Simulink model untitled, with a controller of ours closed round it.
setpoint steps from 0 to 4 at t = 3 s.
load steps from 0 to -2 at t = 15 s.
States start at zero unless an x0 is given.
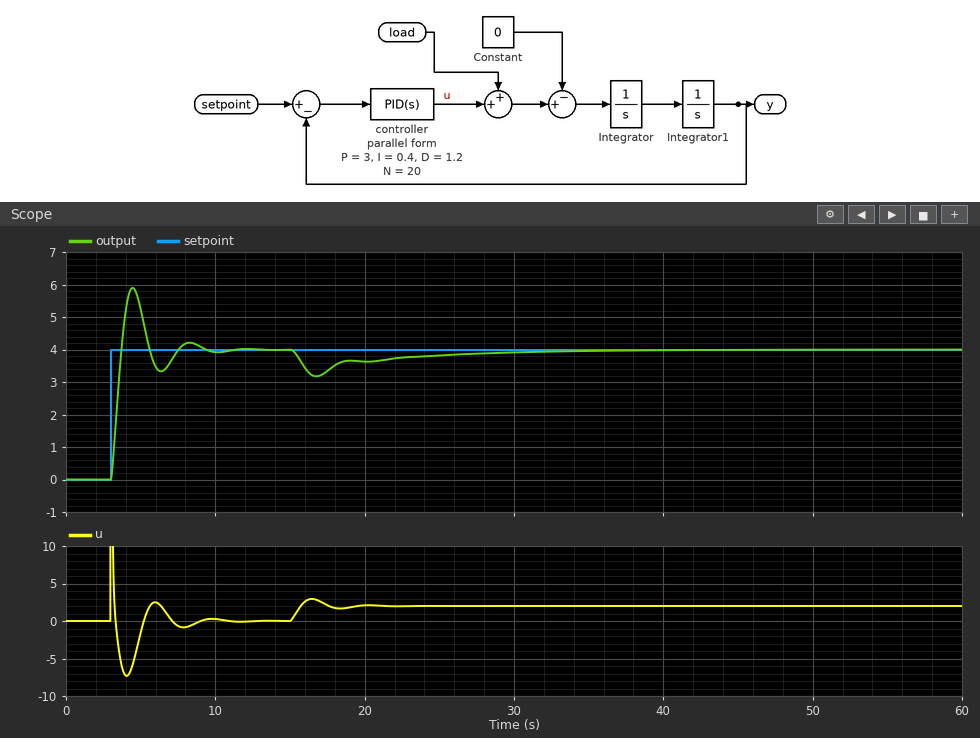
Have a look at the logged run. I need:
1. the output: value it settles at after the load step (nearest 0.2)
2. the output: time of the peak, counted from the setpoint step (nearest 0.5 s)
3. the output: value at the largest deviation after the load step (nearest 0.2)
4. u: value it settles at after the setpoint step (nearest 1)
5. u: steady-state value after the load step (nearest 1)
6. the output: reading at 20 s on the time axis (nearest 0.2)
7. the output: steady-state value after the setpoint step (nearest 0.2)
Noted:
4.0
1.5 s
3.2
0
2
3.6
4.0
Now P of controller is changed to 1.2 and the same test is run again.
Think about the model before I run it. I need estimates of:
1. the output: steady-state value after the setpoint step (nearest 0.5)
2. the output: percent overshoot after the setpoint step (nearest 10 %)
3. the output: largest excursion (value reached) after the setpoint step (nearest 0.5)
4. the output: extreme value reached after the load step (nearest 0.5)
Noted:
4.0
40 %
5.5
2.5
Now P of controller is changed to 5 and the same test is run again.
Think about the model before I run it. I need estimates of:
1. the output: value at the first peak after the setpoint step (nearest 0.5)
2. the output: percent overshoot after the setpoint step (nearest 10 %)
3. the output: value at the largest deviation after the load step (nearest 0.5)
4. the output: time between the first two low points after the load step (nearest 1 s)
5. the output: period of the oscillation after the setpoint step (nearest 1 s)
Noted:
6.0
50 %
3.5
3 s
3 s
